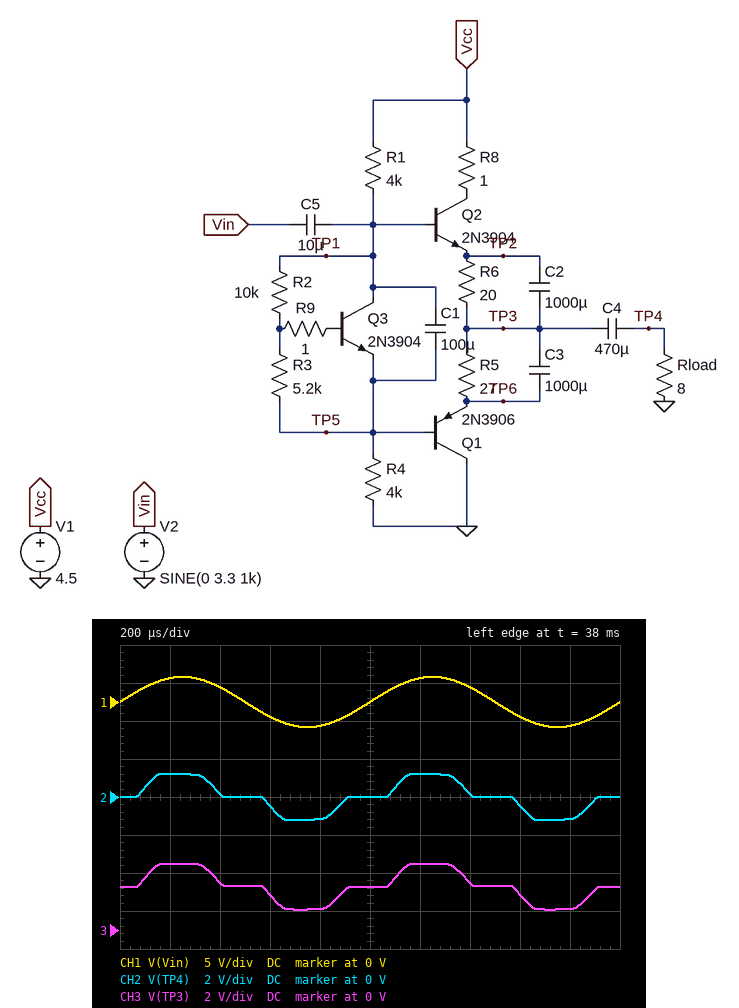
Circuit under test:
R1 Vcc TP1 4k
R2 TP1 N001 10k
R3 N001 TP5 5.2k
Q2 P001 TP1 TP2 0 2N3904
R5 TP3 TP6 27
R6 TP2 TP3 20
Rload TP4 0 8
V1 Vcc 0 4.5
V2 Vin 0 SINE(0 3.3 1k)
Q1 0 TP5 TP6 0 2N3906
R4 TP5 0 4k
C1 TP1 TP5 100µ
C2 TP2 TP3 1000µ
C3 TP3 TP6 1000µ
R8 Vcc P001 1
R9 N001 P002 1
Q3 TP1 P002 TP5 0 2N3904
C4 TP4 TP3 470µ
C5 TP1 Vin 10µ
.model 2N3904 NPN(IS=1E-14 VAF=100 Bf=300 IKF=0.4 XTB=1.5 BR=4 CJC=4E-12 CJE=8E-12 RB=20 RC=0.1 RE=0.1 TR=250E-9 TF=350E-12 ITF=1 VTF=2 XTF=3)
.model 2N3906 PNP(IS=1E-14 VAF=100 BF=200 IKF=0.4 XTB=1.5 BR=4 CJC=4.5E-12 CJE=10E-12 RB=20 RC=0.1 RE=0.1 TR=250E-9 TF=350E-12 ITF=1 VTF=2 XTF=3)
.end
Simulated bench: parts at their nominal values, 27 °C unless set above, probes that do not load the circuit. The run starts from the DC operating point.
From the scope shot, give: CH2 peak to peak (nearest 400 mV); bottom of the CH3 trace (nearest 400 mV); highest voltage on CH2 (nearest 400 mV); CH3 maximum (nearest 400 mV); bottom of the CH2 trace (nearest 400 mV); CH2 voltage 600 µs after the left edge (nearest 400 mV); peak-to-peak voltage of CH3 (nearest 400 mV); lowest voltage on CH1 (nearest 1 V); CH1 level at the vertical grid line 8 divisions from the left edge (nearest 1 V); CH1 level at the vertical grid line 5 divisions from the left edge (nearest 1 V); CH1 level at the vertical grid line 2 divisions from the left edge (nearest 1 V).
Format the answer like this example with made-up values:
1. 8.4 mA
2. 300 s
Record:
1. 2.4 V
2. 1.2 V
3. 1.2 V
4. 3.6 V
5. -1.2 V
6. -400 mV
7. 2.4 V
8. -3 V
9. -2 V
10. 0 V
11. 2 V
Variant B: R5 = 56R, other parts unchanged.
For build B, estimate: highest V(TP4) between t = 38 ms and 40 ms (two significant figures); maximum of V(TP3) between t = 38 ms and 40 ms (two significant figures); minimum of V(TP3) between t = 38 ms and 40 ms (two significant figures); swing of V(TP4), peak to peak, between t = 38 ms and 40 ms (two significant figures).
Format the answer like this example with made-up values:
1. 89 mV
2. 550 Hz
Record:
1. 1.1 V
2. 3.6 V
3. 1.4 V
4. 2.2 V
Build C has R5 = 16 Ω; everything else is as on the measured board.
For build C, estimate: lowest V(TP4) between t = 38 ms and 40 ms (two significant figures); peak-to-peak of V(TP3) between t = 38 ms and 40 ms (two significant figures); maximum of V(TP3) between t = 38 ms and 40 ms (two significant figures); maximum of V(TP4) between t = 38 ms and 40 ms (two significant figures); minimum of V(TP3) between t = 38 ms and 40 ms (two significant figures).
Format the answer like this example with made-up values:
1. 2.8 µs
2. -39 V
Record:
1. -1.3 V
2. 2.6 V
3. 3.4 V
4. 1.3 V
5. 790 mV
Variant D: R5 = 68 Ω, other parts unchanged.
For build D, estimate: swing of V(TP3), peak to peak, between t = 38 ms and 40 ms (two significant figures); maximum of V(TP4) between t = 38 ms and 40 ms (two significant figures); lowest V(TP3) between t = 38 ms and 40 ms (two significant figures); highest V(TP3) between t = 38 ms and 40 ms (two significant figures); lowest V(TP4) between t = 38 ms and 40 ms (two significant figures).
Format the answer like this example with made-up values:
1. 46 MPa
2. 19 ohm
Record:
1. 2.1 V
2. 1.1 V
3. 1.5 V
4. 3.6 V
5. -1.0 V
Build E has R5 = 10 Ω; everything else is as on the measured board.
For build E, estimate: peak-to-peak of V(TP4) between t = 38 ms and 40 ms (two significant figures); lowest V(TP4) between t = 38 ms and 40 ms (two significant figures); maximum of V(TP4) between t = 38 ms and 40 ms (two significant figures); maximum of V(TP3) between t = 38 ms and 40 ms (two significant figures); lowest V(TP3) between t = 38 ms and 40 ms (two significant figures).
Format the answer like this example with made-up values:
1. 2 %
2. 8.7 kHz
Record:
1. 2.8 V
2. -1.4 V
3. 1.4 V
4. 3.4 V
5. 570 mV
